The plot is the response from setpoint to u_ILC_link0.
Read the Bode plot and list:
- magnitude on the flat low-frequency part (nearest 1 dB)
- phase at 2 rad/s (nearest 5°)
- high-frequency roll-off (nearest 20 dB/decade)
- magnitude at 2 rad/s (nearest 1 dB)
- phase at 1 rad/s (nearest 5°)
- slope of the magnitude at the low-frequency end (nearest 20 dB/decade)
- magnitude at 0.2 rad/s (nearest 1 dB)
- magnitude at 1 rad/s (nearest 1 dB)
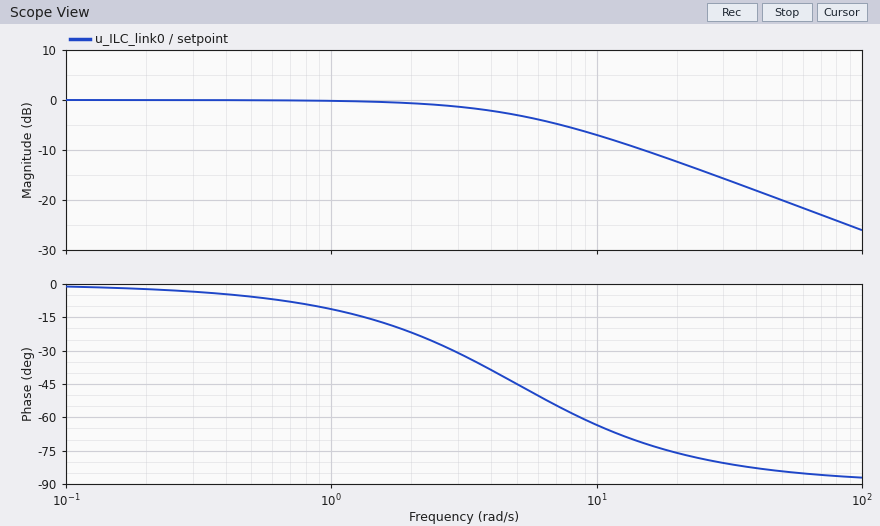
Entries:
0 dB
-20°
-20 dB/decade
-1 dB
-10°
0 dB/decade
0 dB
0 dB
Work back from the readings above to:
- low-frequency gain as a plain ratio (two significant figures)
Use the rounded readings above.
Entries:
1.0
